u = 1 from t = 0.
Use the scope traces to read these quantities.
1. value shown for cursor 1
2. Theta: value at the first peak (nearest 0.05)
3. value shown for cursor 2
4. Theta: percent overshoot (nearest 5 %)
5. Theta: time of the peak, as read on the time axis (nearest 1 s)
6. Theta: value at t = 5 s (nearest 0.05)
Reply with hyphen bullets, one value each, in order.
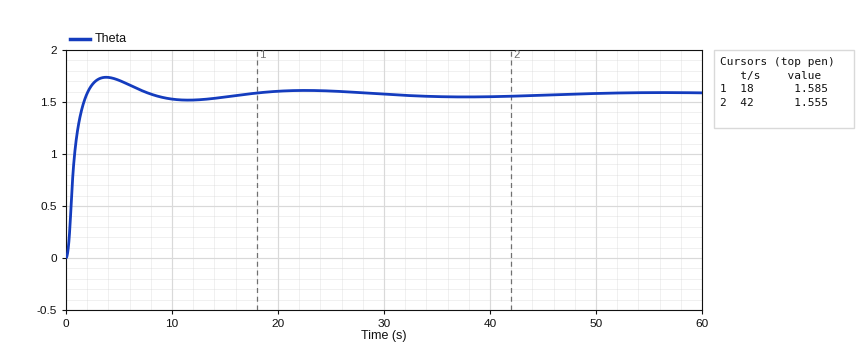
- 1.585
- 1.75
- 1.555
- 10 %
- 4 s
- 1.70
